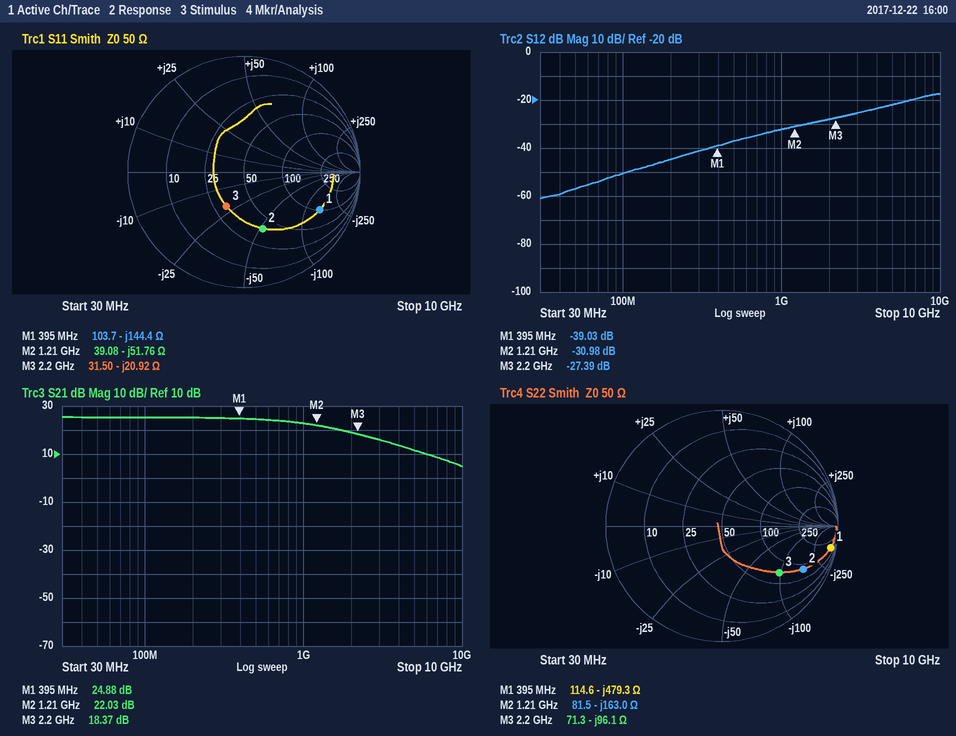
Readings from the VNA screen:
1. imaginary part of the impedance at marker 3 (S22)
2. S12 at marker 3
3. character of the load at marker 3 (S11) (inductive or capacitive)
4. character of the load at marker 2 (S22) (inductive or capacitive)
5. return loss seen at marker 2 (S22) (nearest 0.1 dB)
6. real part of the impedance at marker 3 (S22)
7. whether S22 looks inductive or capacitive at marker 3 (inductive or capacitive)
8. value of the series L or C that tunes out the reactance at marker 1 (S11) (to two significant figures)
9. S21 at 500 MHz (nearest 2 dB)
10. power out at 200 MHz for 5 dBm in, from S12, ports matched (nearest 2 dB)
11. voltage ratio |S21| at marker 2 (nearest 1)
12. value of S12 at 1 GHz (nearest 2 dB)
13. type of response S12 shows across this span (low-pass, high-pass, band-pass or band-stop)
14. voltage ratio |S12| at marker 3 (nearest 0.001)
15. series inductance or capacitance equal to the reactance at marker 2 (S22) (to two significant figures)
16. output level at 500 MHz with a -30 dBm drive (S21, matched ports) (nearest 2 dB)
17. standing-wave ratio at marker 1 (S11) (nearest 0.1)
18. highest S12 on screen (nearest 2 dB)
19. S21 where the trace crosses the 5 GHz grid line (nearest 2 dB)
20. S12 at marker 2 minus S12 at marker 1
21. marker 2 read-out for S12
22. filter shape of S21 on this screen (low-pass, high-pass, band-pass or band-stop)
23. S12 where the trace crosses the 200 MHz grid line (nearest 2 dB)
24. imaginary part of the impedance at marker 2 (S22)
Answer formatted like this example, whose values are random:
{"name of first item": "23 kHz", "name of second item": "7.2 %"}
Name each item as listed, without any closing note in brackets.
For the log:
{"imaginary part of the impedance at marker 3": "-96.1 Ω", "S12 at marker 3": "-27.39 dB", "character of the load at marker 3 (S11)": "capacitive", "character of the load at marker 2 (S22)": "capacitive", "return loss seen at marker 2 (S22)": "2.0 dB", "real part of the impedance at marker 3": "71.3 Ω", "whether S22 looks inductive or capacitive at marker 3": "capacitive", "value of the series L or C that tunes out the reactance at marker 1 (S11)": "58 nH", "S21 at 500 MHz": "24 dB", "power out at 200 MHz for 5 dBm in, from S12, ports matched": "-40 dBm", "voltage ratio |S21| at marker 2": "13", "value of S12 at 1 GHz": "-32 dB", "type of response S12 shows across this span": "high-pass", "voltage ratio |S12| at marker 3": "0.043", "series inductance or capacitance equal to the reactance at marker 2 (S22)": "810 fF", "output level at 500 MHz with a -30 dBm drive (S21, matched ports)": "-6 dBm", "standing-wave ratio at marker 1 (S11)": "6.4", "highest S12 on screen": "-18 dB", "S21 where the trace crosses the 5 GHz grid line": "12 dB", "S12 at marker 2 minus S12 at marker 1": "8.05 dB", "marker 2 read-out for S12": "-30.98 dB", "filter shape of S21 on this screen": "low-pass", "S12 where the trace crosses the 200 MHz grid line": "-44 dB", "imaginary part of the impedance at marker 2": "-163.0 Ω"}
